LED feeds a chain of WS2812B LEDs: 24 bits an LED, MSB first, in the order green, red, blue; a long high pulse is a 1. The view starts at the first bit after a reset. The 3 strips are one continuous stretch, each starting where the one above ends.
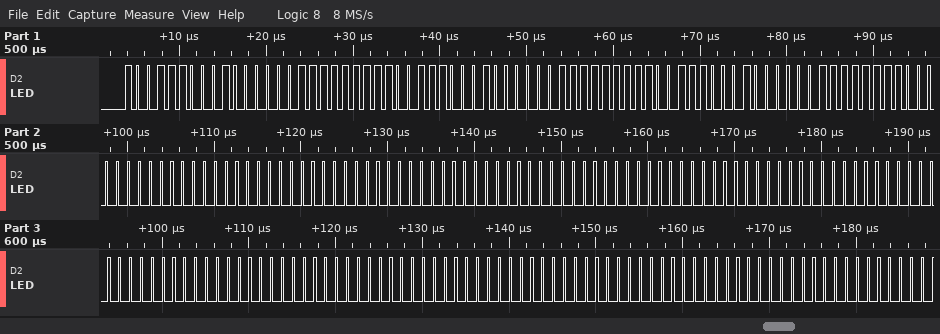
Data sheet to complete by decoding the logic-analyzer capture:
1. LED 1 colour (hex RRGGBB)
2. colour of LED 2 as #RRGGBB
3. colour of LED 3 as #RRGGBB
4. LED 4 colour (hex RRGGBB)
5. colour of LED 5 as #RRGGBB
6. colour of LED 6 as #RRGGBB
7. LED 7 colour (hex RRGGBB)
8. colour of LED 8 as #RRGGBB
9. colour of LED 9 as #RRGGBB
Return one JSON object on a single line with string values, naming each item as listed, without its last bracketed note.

{"LED 1 colour": "#409CFF", "colour of LED 2 as #RRGGBB": "#409CFF", "colour of LED 3 as #RRGGBB": "#409CFF", "LED 4 colour": "#000000", "colour of LED 5 as #RRGGBB": "#000000", "colour of LED 6 as #RRGGBB": "#000000", "LED 7 colour": "#000000", "colour of LED 8 as #RRGGBB": "#000000", "colour of LED 9 as #RRGGBB": "#000000"}
